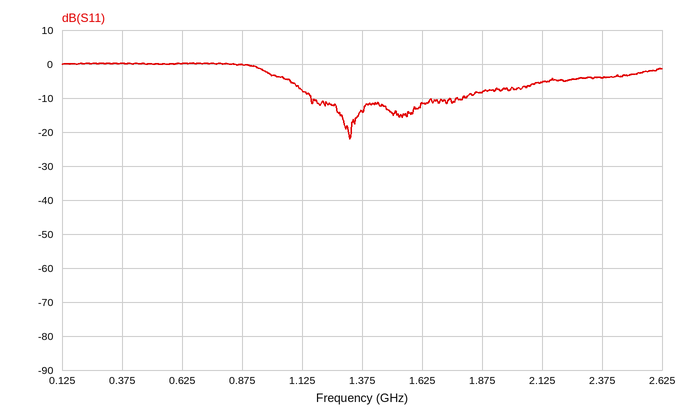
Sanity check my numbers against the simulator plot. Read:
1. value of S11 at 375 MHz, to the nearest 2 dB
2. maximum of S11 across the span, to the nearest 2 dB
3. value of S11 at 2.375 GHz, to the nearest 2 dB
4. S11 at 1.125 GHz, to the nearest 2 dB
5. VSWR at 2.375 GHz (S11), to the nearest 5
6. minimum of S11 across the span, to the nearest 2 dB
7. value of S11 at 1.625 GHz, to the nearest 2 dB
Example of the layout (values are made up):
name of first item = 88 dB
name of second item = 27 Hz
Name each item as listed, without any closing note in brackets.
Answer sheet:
value of S11 at 375 MHz, to the nearest 2 dB = 0 dB
maximum of S11 across the span, to the nearest 2 dB = 0 dB
value of S11 at 2.375 GHz, to the nearest 2 dB = -4 dB
S11 at 1.125 GHz, to the nearest 2 dB = -8 dB
VSWR at 2.375 GHz (S11), to the nearest 5 = 5
minimum of S11 across the span, to the nearest 2 dB = -22 dB
value of S11 at 1.625 GHz, to the nearest 2 dB = -12 dB
